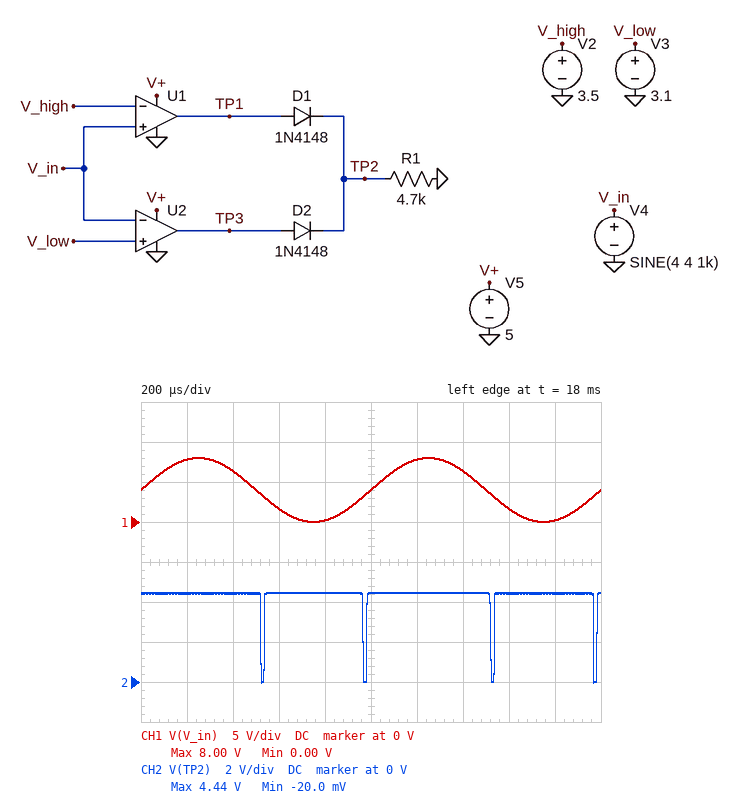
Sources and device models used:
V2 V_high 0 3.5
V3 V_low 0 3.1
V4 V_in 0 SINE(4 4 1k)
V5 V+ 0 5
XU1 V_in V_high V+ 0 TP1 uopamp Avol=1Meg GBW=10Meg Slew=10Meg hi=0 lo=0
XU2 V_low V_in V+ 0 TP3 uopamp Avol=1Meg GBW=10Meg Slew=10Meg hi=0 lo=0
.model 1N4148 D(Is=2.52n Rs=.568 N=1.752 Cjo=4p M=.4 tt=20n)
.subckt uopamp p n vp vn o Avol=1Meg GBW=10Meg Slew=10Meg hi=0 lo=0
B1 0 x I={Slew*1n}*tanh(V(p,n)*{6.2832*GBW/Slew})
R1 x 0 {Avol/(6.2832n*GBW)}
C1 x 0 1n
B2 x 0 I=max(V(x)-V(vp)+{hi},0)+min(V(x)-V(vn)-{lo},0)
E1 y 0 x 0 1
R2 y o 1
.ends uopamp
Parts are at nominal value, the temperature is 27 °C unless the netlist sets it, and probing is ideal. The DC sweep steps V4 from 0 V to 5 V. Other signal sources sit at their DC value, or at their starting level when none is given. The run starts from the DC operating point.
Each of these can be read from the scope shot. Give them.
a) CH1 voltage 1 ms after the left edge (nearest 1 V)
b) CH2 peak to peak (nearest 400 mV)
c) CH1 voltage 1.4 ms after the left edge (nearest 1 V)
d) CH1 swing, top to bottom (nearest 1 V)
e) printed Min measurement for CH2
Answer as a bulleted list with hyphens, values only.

- 4 V
- 4.4 V
- 6 V
- 8 V
- -20.0 mV
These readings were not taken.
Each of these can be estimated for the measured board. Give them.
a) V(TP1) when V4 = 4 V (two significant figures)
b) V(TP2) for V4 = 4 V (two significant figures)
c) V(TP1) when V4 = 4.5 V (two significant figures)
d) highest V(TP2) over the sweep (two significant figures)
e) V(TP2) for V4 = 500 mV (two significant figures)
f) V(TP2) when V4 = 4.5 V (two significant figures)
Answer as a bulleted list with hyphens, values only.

- 5.0 V
- 4.4 V
- 5.0 V
- 4.4 V
- 4.4 V
- 4.4 V
